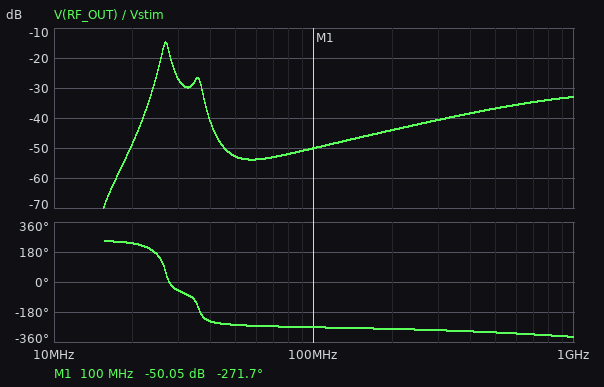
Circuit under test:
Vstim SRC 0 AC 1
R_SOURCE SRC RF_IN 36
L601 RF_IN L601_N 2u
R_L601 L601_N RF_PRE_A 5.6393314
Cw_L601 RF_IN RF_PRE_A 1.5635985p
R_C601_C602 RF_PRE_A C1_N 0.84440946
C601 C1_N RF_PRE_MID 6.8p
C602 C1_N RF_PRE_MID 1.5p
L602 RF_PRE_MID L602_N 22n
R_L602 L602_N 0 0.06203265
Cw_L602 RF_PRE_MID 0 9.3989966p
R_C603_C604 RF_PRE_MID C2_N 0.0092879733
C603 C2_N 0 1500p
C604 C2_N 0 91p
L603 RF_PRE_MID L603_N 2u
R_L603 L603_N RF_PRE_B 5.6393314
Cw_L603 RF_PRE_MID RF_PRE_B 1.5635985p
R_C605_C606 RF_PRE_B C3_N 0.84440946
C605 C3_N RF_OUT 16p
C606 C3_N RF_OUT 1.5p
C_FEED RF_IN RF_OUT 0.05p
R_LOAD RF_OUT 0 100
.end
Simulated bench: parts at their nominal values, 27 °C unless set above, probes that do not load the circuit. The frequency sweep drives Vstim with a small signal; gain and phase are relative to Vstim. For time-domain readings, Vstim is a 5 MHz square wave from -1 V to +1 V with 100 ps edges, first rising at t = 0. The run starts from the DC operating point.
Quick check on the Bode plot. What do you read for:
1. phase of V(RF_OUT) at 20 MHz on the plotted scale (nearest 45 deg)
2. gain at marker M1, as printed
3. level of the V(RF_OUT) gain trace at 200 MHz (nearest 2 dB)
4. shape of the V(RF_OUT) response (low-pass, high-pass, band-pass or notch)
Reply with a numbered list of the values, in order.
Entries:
1. 225 deg
2. -50.05 dB
3. -44 dB
4. band-pass
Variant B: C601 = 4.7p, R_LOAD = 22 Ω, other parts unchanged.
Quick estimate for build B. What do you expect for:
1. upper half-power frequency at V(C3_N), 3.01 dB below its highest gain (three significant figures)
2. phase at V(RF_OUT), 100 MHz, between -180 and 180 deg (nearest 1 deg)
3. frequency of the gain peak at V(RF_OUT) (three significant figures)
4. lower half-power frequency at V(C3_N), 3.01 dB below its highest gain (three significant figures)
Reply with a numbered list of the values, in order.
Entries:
1. 28.0 MHz
2. 89 deg
3. 27.5 MHz
4. 26.9 MHz
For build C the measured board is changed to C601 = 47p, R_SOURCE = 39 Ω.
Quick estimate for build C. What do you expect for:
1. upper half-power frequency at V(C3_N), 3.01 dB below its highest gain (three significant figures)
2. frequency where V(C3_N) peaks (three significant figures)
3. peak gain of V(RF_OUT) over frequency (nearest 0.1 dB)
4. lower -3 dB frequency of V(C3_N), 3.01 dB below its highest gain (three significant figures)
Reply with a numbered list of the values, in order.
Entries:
1. 27.8 MHz
2. 27.1 MHz
3. -12.4 dB
4. 26.2 MHz
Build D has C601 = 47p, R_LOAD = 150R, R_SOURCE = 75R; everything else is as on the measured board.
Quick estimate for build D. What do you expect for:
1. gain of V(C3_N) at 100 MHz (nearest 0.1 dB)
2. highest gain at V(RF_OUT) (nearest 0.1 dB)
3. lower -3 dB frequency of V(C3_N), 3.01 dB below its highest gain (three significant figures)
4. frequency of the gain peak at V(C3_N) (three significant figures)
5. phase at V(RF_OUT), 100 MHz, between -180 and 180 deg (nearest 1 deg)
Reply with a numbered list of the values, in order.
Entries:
1. -46.7 dB
2. -11.0 dB
3. 26.3 MHz
4. 27.0 MHz
5. 87 deg
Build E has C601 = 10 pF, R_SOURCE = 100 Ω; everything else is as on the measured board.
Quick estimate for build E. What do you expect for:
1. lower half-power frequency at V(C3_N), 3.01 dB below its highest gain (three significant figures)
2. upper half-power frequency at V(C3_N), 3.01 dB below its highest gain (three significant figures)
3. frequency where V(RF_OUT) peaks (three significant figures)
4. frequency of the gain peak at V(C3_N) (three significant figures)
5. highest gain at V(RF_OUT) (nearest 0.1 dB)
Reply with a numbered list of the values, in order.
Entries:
1. 25.9 MHz
2. 27.7 MHz
3. 26.8 MHz
4. 26.8 MHz
5. -10.8 dB
